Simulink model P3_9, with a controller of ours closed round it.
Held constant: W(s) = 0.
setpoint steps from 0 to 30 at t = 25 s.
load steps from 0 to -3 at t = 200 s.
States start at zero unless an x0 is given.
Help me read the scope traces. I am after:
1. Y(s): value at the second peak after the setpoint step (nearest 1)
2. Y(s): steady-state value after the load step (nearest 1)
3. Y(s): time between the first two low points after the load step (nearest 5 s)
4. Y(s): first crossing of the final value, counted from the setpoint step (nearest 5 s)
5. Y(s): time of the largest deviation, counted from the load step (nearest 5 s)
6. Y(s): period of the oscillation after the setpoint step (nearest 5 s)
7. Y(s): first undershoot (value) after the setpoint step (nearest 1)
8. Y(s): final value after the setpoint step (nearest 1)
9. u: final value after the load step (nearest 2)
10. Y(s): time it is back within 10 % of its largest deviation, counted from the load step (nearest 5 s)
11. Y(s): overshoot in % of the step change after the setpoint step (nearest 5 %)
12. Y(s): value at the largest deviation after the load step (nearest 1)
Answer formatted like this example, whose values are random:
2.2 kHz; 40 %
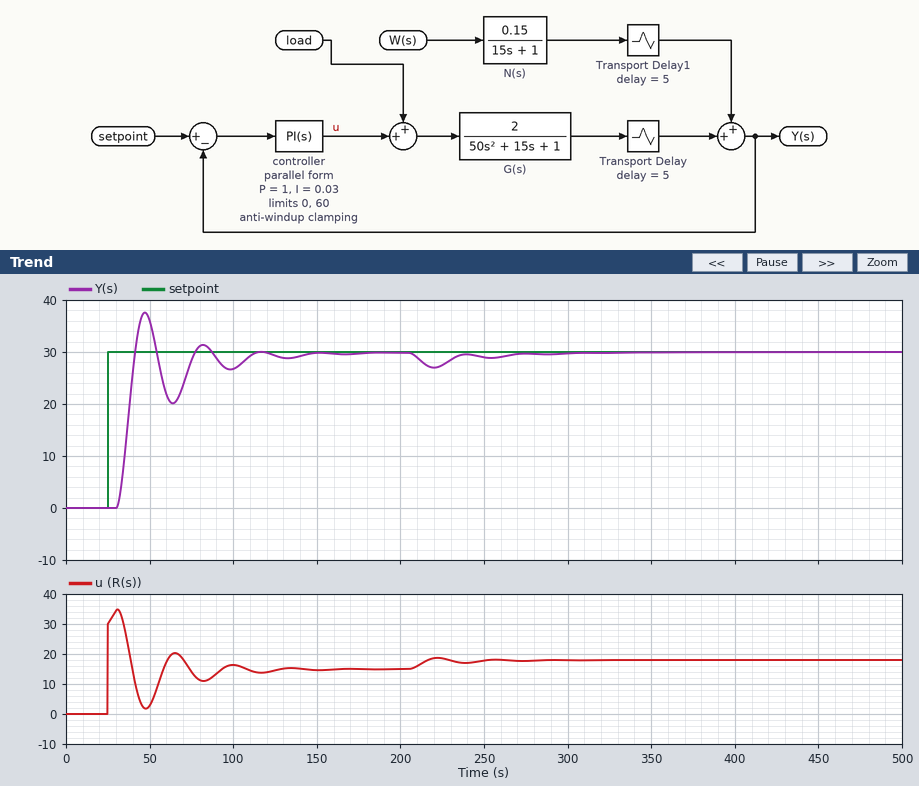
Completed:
31; 30; 35 s; 15 s; 20 s; 35 s; 20; 30; 18; 100 s; 25 %; 27
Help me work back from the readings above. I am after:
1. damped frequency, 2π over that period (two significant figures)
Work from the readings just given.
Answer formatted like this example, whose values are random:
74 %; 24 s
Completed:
0.18 rad/s
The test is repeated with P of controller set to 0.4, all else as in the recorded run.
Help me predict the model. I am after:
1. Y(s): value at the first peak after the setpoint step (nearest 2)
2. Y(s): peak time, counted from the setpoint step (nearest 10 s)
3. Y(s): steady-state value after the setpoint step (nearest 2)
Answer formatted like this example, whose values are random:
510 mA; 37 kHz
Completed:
32; 40 s; 30
